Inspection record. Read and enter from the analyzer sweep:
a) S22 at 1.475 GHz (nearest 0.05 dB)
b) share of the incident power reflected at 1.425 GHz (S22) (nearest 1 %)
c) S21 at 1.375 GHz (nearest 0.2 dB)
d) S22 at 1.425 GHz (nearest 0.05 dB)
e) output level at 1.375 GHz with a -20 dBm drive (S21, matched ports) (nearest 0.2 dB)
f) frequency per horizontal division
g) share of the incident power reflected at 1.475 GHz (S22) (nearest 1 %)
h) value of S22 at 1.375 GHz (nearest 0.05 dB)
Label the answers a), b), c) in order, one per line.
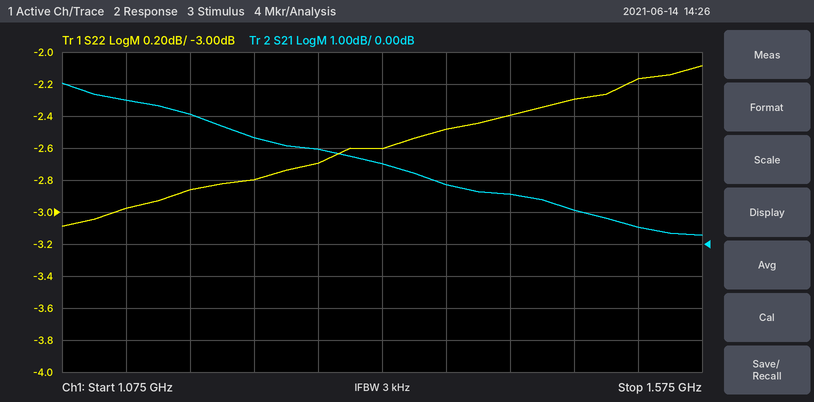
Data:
a) -2.30 dB
b) 58 %
c) 1.8 dB
d) -2.40 dB
e) -18.2 dBm
f) 50 MHz
g) 59 %
h) -2.50 dB
